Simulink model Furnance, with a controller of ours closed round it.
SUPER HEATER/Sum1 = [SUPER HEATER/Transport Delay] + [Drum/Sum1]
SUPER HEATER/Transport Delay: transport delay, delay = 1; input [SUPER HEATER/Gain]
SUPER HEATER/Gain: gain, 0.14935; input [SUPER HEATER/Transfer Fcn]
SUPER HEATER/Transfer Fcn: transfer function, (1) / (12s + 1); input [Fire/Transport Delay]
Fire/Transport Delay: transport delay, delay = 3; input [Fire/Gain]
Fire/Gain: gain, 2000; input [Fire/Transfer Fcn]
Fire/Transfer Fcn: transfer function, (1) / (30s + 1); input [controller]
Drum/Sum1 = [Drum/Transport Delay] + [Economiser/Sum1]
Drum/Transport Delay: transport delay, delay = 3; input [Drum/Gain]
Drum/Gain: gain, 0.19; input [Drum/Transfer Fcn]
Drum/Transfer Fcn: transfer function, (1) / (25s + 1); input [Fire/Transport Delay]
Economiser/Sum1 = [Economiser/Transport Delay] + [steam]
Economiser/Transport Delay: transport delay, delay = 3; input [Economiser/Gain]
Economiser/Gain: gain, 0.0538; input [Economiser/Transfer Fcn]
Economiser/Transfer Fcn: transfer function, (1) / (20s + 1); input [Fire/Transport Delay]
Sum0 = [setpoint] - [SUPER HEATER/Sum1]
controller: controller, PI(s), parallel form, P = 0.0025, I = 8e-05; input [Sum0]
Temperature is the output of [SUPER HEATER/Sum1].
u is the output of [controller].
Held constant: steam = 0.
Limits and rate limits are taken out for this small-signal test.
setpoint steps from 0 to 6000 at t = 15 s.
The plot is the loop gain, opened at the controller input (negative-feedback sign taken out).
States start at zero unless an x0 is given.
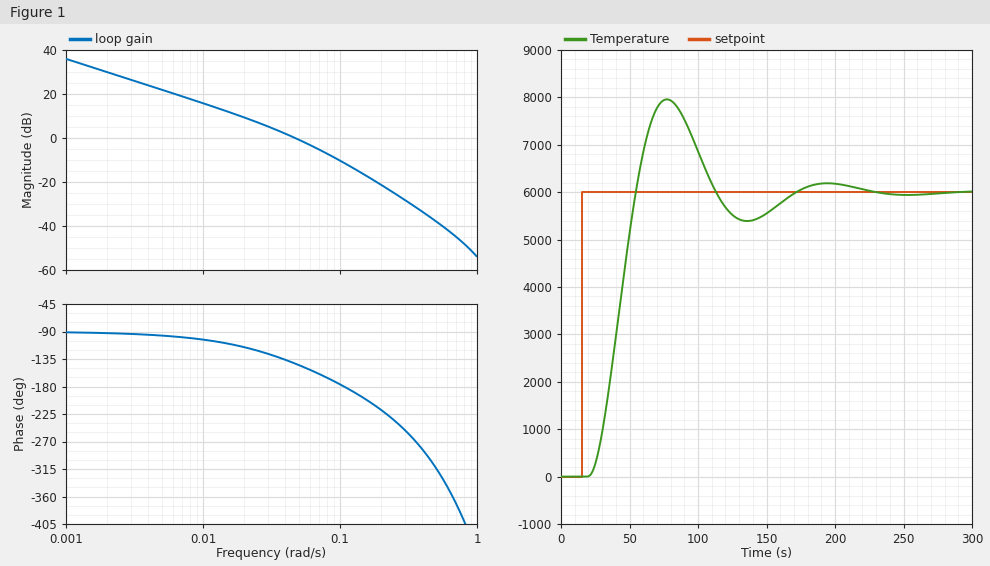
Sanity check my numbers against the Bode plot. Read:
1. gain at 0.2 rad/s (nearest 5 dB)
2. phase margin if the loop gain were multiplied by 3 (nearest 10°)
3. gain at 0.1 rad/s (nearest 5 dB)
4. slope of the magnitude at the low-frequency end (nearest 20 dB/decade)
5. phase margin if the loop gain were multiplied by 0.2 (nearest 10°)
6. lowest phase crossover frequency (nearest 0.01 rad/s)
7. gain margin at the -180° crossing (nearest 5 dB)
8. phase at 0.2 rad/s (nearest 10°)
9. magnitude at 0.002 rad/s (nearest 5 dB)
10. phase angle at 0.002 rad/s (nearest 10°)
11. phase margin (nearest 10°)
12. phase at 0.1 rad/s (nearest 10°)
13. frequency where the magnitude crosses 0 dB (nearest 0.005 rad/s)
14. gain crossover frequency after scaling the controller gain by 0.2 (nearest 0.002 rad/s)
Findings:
-20 dB
10°
-10 dB
-20 dB/decade
70°
0.11 rad/s
10 dB
-220°
30 dB
-90°
40°
-180°
0.045 rad/s
0.012 rad/s
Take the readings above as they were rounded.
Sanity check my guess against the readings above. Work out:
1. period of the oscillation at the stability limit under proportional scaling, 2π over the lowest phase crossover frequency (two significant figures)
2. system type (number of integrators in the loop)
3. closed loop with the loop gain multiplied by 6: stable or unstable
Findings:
57 s
1
unstable
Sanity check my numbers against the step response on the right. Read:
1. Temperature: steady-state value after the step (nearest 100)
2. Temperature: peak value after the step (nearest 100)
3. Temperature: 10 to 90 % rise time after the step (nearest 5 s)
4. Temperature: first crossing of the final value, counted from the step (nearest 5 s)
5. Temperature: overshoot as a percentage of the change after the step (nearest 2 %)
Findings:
6000
8000
25 s
40 s
32 %
